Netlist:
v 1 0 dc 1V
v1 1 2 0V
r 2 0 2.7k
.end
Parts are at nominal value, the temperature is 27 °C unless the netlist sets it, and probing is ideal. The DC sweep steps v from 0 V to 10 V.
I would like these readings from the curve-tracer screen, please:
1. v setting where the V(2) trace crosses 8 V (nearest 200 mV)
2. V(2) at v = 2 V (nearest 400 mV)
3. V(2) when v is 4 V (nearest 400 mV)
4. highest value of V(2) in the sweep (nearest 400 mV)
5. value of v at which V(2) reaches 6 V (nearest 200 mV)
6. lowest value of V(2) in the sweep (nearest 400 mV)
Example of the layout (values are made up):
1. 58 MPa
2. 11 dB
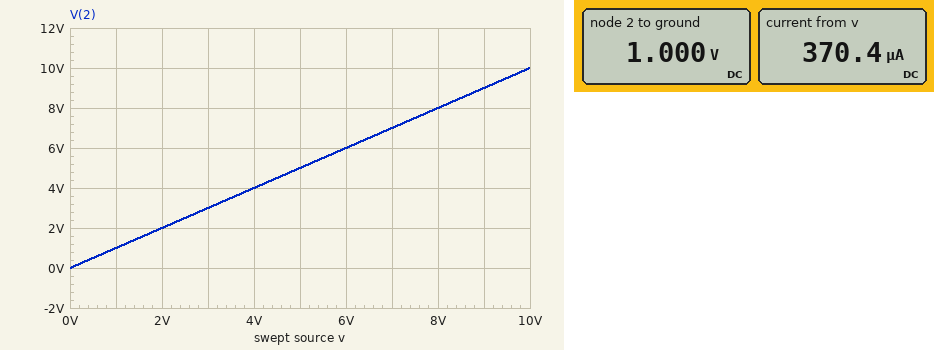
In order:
1. 8.0 V
2. 2.0 V
3. 4.0 V
4. 10.0 V
5. 6.0 V
6. 0 V
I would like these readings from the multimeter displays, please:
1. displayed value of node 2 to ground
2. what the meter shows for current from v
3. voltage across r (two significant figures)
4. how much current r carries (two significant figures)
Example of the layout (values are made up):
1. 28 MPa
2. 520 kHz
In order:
1. 1.000 V
2. 370.4 µA
3. 1.0 V
4. 370 µA
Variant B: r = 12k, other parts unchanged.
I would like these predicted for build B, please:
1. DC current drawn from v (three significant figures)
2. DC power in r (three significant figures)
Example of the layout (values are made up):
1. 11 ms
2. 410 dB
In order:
1. 83.3 µA
2. 83.3 µW
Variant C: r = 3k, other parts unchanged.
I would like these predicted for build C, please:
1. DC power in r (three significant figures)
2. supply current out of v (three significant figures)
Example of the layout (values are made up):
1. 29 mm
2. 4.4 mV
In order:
1. 333 µW
2. 333 µA
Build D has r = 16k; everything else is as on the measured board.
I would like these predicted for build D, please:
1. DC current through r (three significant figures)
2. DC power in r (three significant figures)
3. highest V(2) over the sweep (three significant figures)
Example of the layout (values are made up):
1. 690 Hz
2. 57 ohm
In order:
1. 62.5 µA
2. 62.5 µW
3. 10.0 V
